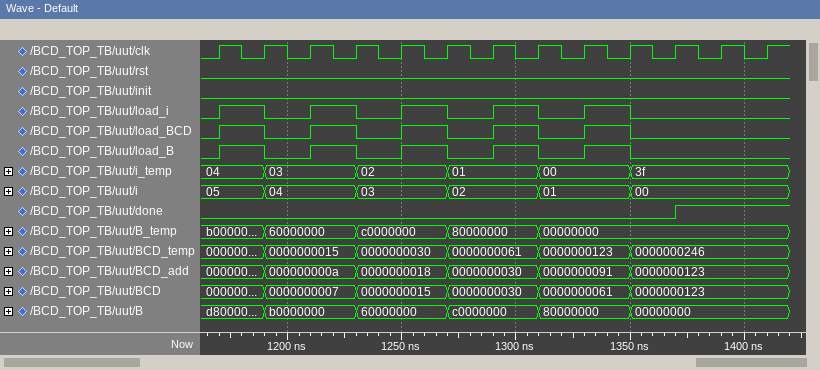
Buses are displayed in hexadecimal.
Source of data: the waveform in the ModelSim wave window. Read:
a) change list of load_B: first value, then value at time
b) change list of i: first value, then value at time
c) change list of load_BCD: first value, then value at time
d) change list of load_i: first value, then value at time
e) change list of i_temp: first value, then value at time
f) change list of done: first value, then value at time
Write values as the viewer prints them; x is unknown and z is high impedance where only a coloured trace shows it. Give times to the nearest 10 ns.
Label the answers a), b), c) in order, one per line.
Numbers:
a) 0, 1 at 1170 ns, 0 at 1190 ns, 1 at 1210 ns, 0 at 1230 ns, 1 at 1250 ns, 0 at 1270 ns, 1 at 1290 ns, 0 at 1310 ns, 1 at 1330 ns, 0 at 1350 ns
b) 05, 04 at 1190 ns, 03 at 1230 ns, 02 at 1270 ns, 01 at 1310 ns, 00 at 1350 ns
c) 0, 1 at 1170 ns, 0 at 1190 ns, 1 at 1210 ns, 0 at 1230 ns, 1 at 1250 ns, 0 at 1270 ns, 1 at 1290 ns, 0 at 1310 ns, 1 at 1330 ns, 0 at 1350 ns
d) 0, 1 at 1170 ns, 0 at 1190 ns, 1 at 1210 ns, 0 at 1230 ns, 1 at 1250 ns, 0 at 1270 ns, 1 at 1290 ns, 0 at 1310 ns, 1 at 1330 ns, 0 at 1350 ns
e) 04, 03 at 1190 ns, 02 at 1230 ns, 01 at 1270 ns, 00 at 1310 ns, 3f at 1350 ns
f) 0, 1 at 1370 ns
